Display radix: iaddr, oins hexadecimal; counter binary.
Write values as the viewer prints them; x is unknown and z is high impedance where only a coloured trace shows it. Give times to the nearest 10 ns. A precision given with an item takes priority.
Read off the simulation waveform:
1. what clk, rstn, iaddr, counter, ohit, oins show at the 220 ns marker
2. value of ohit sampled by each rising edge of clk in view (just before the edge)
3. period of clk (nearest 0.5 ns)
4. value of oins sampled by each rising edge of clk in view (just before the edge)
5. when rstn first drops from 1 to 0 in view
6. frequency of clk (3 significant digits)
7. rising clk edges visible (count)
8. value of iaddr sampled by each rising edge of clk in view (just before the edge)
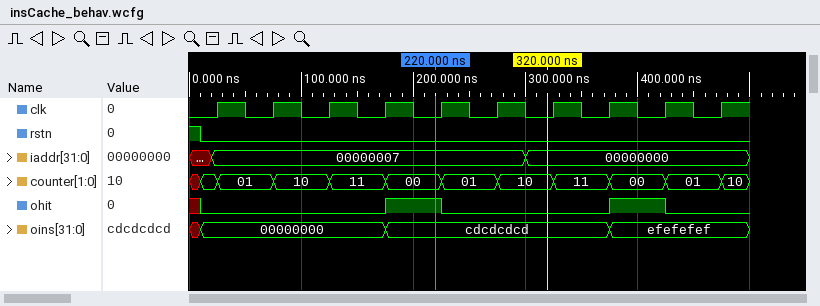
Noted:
clk=0, rstn=0, iaddr=00000007, counter=00, ohit=1, oins=cdcdcdcd
0 0 0 0 1 0 0 0 1 0
50 ns
00000000, 00000000, 00000000, 00000000, cdcdcdcd, cdcdcdcd, cdcdcdcd, cdcdcdcd, efefefef, efefefef
10 ns
20.0 MHz
10
00000007, 00000007, 00000007, 00000007, 00000007, 00000007, 00000000, 00000000, 00000000, 00000000
